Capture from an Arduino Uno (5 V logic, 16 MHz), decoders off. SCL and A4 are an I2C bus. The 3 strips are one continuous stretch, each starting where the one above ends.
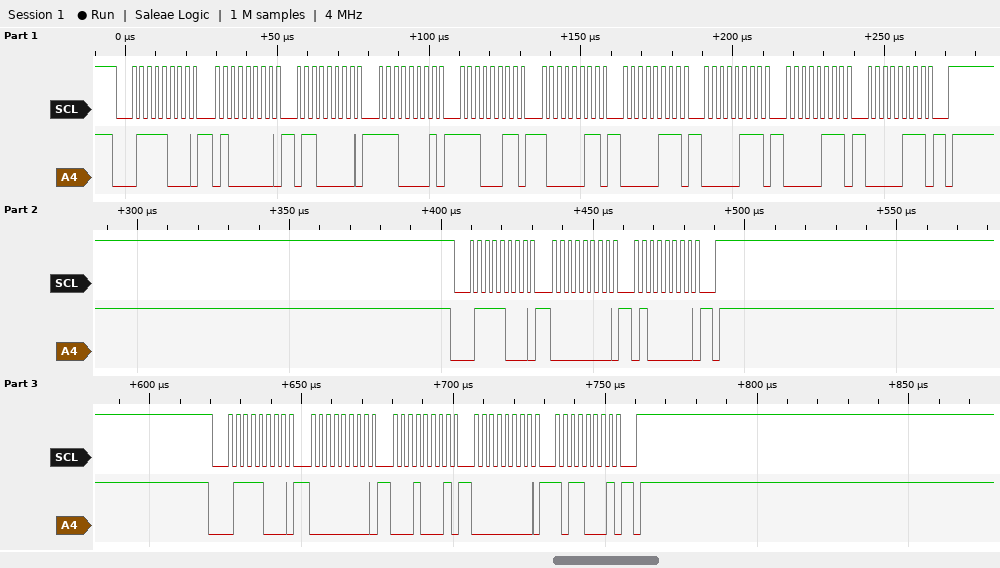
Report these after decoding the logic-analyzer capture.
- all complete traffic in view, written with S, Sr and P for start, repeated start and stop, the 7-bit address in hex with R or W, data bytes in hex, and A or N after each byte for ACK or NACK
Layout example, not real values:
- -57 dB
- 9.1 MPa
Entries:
- S 3CW A 40 A 60 A E1 A E3 A 83 A 07 A 07 A 07 A 07 A P S 3CW A 00 A 40 A P S 3CW A 00 A 11 A 00 A B1 A P
